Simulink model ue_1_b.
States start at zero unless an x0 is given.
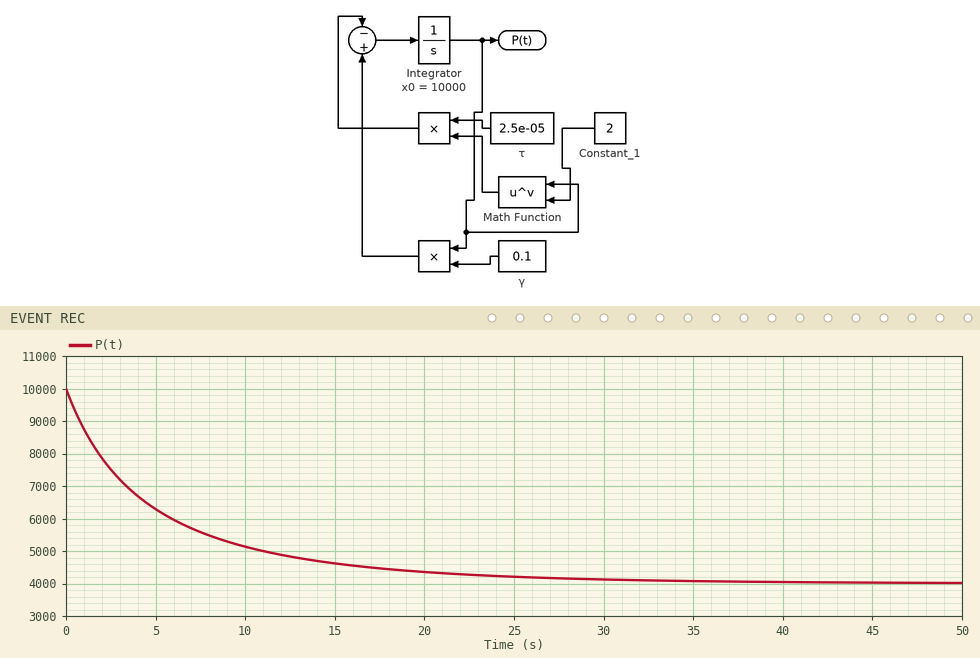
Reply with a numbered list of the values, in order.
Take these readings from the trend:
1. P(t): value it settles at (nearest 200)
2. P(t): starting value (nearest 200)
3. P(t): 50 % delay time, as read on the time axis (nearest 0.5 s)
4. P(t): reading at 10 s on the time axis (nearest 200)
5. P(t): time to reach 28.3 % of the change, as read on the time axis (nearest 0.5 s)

1. 4000
2. 10000
3. 3.5 s
4. 5200
5. 1.5 s
